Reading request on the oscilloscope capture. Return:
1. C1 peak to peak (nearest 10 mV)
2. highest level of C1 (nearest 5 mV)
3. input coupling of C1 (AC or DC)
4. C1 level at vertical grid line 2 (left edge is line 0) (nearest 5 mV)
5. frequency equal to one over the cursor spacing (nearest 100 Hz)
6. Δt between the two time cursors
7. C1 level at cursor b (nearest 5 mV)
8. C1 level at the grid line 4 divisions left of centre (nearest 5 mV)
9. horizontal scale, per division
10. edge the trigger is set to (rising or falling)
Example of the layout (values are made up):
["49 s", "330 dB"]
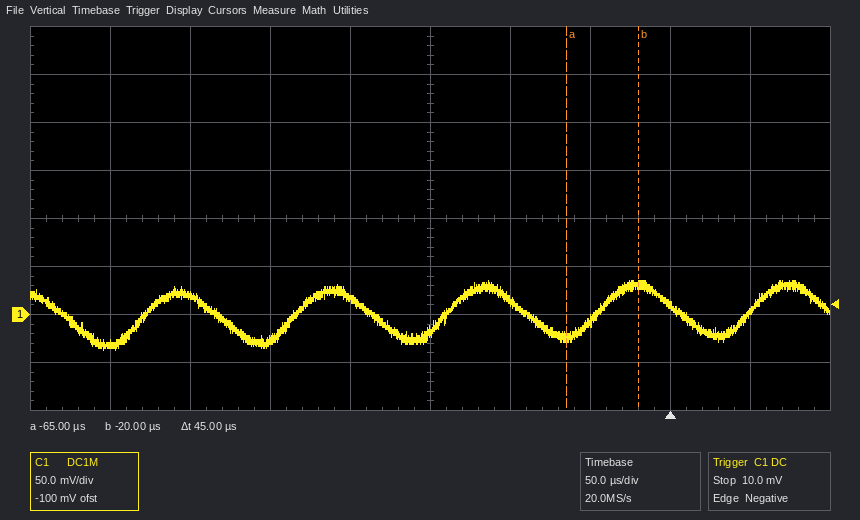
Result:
["70 mV", "35 mV", "DC", "20 mV", "22.2 kHz", "45 µs", "30 mV", "-30 mV", "50 µs", "falling"]
